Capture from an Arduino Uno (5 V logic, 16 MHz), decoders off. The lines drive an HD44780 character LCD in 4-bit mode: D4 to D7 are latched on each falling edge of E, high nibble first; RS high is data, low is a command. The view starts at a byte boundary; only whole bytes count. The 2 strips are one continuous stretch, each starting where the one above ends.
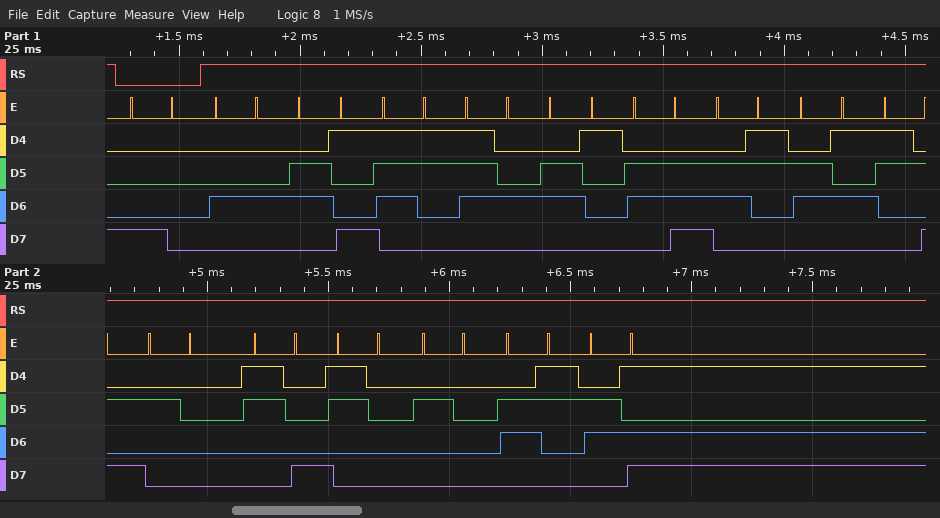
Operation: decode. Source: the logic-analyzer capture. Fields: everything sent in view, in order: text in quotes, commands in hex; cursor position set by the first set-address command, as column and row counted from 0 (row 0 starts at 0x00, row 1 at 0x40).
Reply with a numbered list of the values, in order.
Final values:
1. 0x80 "Distance: 80 cm"
2. column 0, row 0
